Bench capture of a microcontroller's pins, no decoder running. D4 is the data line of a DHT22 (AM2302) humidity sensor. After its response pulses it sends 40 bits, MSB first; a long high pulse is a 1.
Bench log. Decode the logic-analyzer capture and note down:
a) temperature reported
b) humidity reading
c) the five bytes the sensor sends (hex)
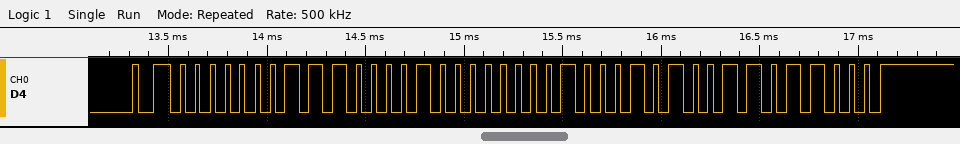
27.6 °C
45.0 %
01 C2 01 14 D8
